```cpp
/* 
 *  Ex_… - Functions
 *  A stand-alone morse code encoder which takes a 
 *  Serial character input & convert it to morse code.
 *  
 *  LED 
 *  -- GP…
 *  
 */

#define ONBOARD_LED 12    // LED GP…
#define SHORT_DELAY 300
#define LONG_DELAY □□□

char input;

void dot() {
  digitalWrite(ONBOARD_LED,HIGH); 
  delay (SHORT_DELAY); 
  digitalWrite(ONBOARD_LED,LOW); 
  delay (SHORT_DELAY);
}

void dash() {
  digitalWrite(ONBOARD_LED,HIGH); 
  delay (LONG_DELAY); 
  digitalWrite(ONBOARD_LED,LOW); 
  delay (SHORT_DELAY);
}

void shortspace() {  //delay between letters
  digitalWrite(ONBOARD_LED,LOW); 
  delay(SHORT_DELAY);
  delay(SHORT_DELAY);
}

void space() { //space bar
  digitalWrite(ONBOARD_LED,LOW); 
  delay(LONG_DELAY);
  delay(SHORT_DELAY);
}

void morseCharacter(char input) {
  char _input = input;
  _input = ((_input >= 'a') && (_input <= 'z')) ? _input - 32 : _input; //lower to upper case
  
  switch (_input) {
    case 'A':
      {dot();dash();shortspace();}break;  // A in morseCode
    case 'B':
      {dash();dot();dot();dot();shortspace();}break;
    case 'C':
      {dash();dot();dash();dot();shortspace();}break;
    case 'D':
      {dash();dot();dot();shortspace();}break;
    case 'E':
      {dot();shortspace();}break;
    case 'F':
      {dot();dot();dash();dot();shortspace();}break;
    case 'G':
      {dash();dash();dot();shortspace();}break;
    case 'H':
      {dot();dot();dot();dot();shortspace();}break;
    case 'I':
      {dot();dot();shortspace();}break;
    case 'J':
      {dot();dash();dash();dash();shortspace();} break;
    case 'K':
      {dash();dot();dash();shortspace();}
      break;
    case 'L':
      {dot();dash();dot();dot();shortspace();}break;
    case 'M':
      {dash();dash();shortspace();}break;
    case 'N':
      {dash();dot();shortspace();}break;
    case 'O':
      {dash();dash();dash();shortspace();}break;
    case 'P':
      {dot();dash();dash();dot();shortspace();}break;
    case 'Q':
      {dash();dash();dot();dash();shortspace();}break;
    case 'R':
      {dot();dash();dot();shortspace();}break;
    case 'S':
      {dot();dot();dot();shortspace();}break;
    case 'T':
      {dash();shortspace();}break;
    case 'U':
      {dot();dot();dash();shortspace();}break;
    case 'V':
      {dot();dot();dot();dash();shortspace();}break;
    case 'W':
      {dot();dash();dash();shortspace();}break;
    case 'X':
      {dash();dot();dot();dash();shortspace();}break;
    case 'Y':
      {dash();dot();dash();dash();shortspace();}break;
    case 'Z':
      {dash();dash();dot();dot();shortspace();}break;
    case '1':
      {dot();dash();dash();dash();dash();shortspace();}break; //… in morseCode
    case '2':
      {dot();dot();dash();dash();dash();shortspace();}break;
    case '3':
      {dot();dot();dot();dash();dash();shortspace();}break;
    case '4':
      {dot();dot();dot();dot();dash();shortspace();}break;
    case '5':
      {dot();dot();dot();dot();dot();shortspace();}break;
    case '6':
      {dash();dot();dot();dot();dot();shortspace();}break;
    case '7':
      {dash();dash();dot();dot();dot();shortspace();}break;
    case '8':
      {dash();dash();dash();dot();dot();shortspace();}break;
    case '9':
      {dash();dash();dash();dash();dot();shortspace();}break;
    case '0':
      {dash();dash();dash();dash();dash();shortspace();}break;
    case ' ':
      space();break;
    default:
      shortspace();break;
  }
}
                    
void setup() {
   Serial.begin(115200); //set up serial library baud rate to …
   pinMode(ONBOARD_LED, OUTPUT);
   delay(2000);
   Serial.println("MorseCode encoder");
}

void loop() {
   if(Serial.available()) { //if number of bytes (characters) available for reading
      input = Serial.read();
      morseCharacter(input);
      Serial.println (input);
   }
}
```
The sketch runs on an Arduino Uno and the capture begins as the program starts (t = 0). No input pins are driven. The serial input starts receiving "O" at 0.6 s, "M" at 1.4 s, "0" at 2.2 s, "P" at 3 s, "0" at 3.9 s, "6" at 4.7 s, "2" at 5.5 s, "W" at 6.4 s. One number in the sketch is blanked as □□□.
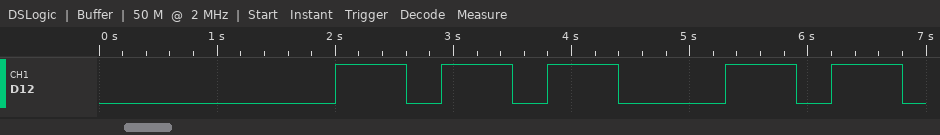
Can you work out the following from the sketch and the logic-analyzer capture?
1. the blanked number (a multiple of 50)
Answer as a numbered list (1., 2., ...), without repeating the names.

1. 600
